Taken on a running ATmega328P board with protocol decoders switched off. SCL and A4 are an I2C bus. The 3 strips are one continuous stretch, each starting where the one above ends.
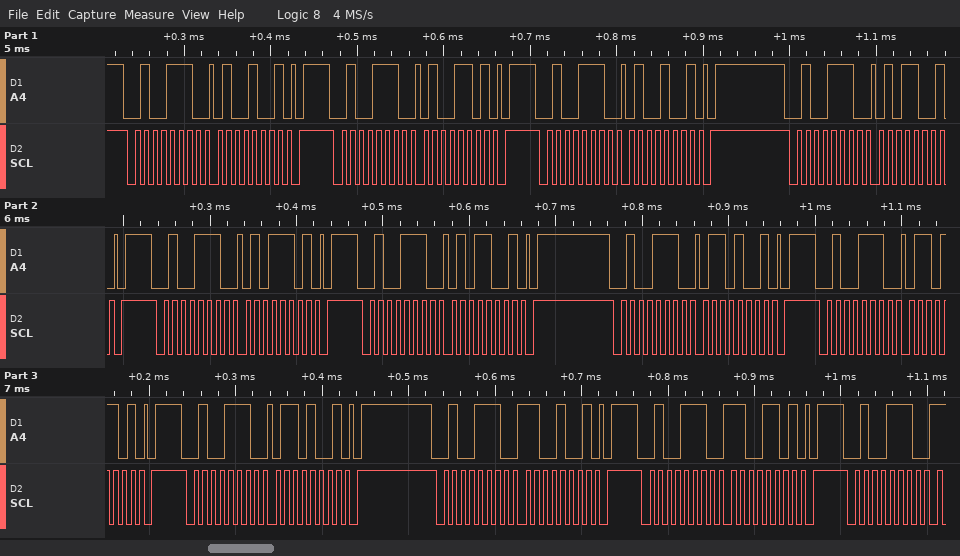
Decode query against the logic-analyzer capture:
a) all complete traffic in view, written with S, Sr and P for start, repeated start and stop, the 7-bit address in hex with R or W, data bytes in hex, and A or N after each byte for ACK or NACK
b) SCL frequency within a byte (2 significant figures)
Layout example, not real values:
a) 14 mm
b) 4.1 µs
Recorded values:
a) S 27W A 49 A P S 27W A 4D A P S 27W A 49 A P S 27W A 59 A P S 27W A 5D A P S 27W A 59 A P S 27W A 69 A P S 27W A 6D A P S 27W A 69 A P S 27W A C9 A P S 27W A CD A P S 27W A
b) 100 kHz
